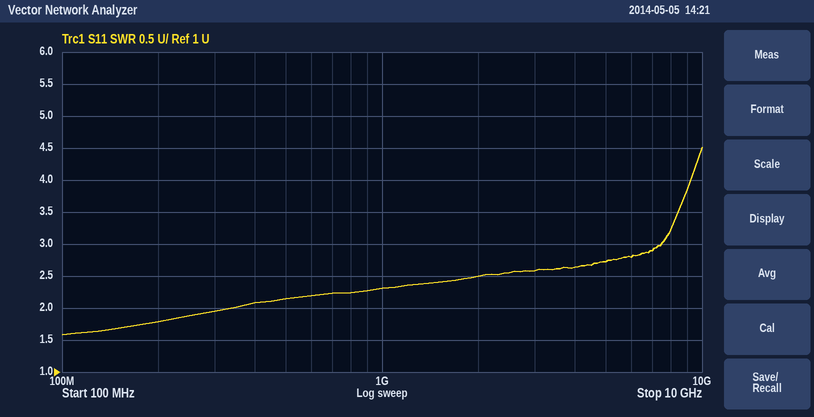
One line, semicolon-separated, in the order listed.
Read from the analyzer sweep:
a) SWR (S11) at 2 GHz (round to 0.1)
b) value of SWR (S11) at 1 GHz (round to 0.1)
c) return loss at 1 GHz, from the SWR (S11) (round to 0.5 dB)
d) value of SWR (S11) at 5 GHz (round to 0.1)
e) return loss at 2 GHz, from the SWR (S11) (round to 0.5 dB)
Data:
2.5; 2.3; 8.0 dB; 2.7; 7.5 dB
